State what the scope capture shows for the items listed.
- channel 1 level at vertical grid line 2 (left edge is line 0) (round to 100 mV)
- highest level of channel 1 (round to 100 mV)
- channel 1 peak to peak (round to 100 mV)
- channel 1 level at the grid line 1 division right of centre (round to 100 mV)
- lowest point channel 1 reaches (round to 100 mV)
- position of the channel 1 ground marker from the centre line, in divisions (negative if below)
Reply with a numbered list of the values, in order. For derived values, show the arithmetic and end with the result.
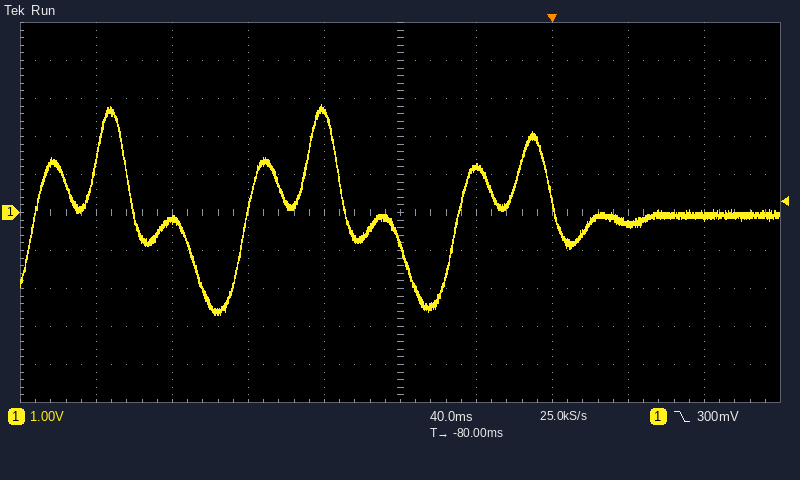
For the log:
1. -200 mV
2. 2.8 V
3. 2.8 V − (-2.7 V) = 5.5 V
4. 1.2 V
5. -2.7 V
6. 0.0 div
